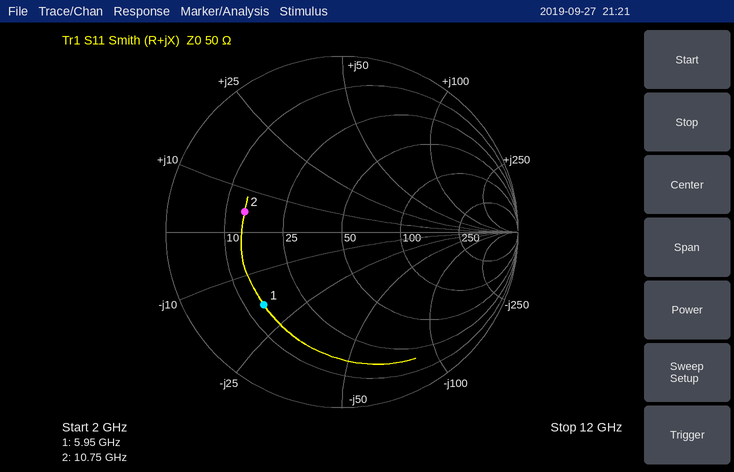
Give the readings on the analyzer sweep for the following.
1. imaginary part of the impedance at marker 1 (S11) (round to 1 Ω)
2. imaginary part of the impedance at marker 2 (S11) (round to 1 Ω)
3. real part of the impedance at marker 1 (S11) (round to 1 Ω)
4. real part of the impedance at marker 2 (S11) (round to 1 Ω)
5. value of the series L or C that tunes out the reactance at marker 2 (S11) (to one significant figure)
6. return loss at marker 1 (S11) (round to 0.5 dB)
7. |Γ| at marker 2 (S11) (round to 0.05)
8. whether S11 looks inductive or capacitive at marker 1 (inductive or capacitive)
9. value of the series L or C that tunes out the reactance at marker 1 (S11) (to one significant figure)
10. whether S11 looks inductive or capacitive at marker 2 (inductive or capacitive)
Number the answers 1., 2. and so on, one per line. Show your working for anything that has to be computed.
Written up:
1. -18 Ω
2. +5 Ω
3. 14 Ω
4. 14 Ω
5. C = 1/(2π × 10.75 GHz × 5 Ω) ≈ 3 pF
6. 4.5 dB
7. 0.55
8. capacitive
9. L = 18 Ω/(2π × 5.95 GHz) ≈ 481 pH, so 500 pH to one significant figure
10. inductive
